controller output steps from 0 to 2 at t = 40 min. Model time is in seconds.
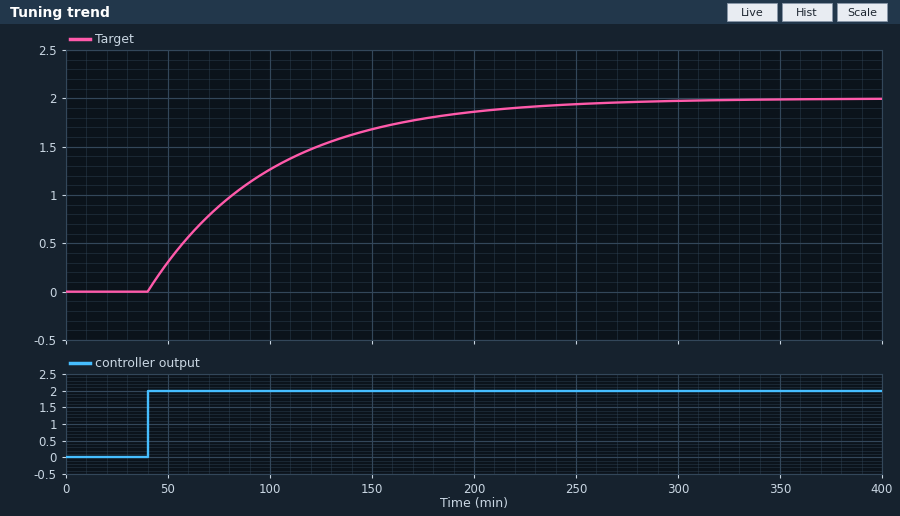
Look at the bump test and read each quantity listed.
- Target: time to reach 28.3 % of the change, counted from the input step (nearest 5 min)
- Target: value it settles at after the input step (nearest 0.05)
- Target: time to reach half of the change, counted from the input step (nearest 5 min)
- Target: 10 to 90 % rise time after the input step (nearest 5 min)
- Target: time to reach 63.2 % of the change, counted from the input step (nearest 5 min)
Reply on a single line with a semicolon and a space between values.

20 min; 2.00; 40 min; 130 min; 60 min
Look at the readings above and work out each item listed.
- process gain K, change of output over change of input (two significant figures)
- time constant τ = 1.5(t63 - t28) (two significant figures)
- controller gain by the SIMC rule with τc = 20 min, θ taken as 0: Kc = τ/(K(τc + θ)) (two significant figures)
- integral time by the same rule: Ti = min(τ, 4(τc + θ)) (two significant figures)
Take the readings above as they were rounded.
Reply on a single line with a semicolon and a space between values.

1.0; 60 min; 3.0; 60 min
